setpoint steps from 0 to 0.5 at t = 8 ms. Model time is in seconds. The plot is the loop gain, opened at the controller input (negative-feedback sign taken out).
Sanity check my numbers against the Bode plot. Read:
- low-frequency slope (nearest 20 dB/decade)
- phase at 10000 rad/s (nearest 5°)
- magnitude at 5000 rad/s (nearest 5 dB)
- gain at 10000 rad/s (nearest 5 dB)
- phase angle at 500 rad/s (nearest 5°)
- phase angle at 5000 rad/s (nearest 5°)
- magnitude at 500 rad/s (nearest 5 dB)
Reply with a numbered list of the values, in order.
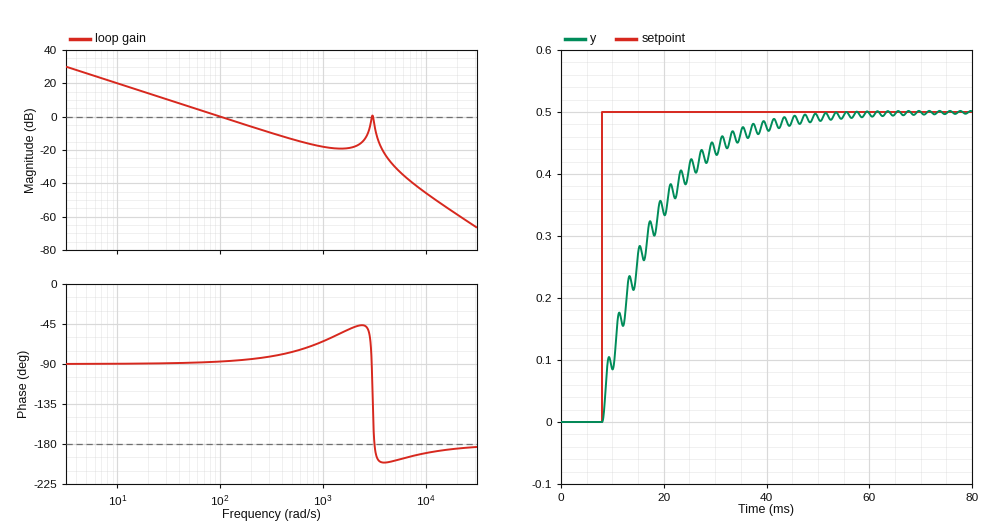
1. -20 dB/decade
2. -190°
3. -30 dB
4. -45 dB
5. -75°
6. -200°
7. -15 dB
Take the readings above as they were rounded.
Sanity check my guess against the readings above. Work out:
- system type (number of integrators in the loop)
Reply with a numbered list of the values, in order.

1. 1
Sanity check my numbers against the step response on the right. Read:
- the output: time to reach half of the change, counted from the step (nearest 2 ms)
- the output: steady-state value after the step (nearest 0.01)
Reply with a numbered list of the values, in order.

1. 6 ms
2. 0.50
